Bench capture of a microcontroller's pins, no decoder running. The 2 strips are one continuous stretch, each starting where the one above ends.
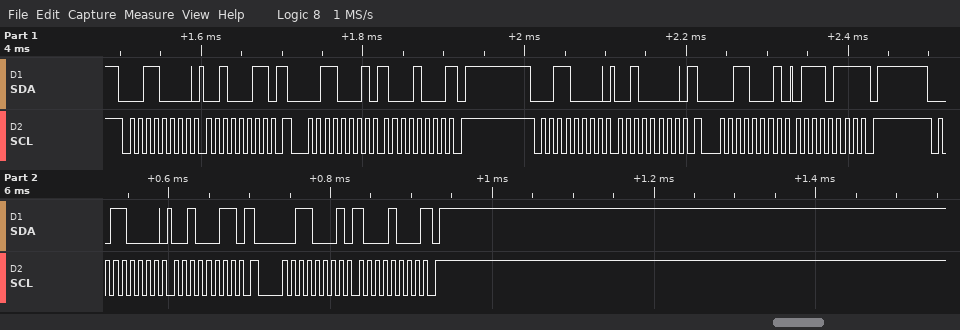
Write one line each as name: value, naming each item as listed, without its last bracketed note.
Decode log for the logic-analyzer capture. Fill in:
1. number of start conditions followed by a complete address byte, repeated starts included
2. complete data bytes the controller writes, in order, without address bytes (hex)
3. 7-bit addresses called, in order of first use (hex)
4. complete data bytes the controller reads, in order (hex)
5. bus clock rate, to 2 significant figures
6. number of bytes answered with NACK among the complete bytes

number of start conditions followed by a complete address byte, repeated starts included: 6
complete data bytes the controller writes, in order, without address bytes: 23 20 23
7-bit addresses called, in order of first use: 0x18
complete data bytes the controller reads, in order: 88 77 88
bus clock rate, to 2 significant figures: 100 kHz
number of bytes answered with NACK among the complete bytes: 3
